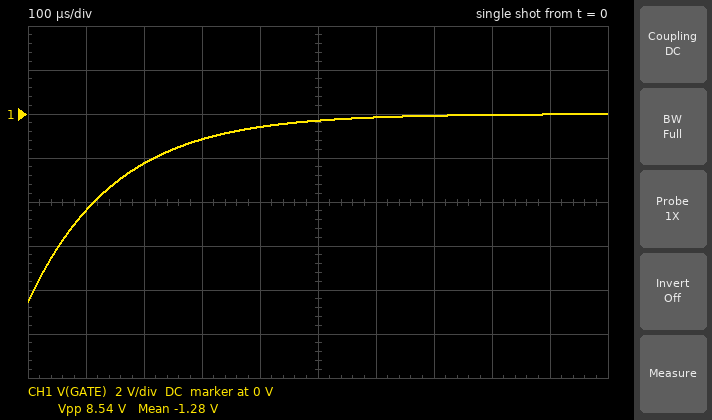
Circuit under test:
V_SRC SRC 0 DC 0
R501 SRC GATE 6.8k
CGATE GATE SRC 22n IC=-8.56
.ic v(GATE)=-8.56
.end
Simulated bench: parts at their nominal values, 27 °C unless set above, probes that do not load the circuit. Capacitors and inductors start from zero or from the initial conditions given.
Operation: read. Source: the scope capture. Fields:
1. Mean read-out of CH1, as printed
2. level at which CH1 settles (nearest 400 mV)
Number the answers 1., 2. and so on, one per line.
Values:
1. -1.28 V
2. 0 V
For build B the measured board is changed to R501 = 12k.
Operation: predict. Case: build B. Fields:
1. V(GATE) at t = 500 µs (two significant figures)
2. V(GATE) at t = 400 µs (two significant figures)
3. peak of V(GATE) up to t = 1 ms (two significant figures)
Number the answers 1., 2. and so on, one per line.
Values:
1. -1.3 V
2. -1.9 V
3. -190 mV
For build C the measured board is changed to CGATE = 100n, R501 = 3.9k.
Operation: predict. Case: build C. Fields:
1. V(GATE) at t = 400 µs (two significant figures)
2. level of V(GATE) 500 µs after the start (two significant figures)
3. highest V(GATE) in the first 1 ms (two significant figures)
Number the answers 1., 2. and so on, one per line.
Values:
1. -3.1 V
2. -2.4 V
3. -660 mV
